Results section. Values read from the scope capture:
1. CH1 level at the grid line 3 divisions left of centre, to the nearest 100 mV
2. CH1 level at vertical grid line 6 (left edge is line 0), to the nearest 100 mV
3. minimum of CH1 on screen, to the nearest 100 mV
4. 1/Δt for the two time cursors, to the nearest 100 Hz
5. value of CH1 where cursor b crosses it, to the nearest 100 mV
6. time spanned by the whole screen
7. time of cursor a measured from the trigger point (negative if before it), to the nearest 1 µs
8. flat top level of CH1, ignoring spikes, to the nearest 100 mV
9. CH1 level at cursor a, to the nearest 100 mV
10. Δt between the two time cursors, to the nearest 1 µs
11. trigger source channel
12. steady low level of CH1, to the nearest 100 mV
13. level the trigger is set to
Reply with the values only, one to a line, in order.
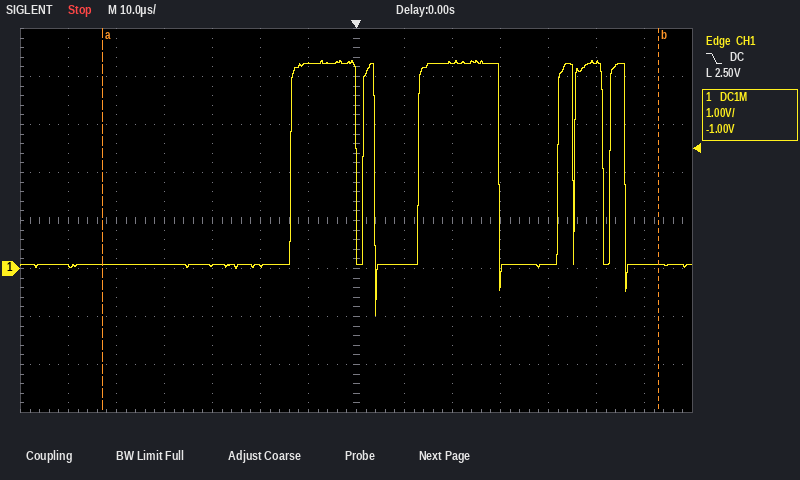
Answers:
100 mV
4.3 V
-1.0 V
8.6 kHz
100 mV
140 µs
-53 µs
4.3 V
100 mV
116 µs
CH1
100 mV
2.50 V
